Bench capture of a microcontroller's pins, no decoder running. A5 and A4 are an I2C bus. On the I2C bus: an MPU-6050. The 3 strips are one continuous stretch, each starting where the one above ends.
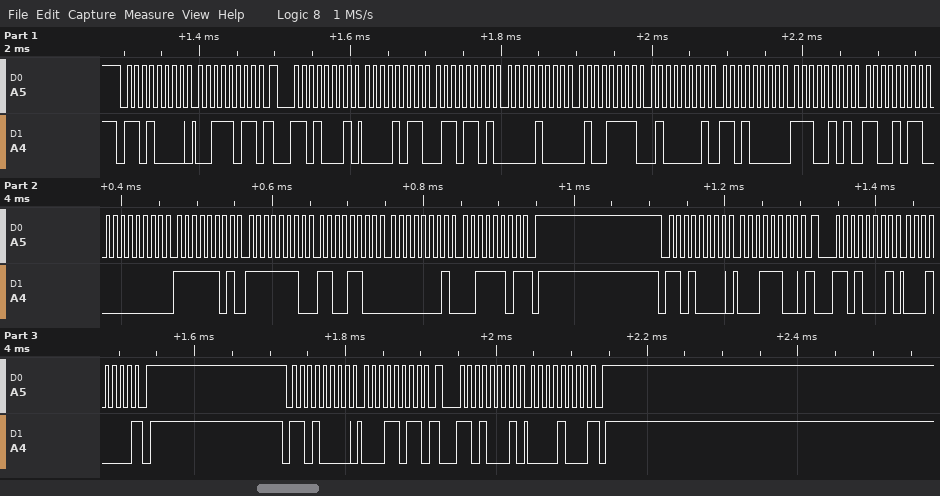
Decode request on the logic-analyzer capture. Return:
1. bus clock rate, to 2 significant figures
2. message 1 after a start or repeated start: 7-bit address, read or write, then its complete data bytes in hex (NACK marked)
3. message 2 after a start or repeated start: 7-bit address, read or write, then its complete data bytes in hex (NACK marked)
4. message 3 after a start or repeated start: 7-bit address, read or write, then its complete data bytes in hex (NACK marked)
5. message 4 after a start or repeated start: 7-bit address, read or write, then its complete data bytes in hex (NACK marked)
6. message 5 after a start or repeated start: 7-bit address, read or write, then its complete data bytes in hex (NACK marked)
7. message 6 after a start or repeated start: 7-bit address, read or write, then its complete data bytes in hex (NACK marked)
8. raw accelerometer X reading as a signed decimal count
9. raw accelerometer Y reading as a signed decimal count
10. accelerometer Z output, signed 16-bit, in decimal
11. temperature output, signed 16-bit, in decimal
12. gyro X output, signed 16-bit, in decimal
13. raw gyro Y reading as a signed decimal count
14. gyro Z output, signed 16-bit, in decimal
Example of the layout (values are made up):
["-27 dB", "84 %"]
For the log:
["100 kHz", "0x68 write: 3B", "0x68 read: 0B 6D 08 4F 41 D0 E5 CB 00 FD FE CC 01 3D NACK", "0x68 write: 1C", "0x68 read: 10 NACK", "0x68 write: 1B", "0x68 read: 08 NACK", "2925", "2127", "16848", "-6709", "253", "-308", "317"]
